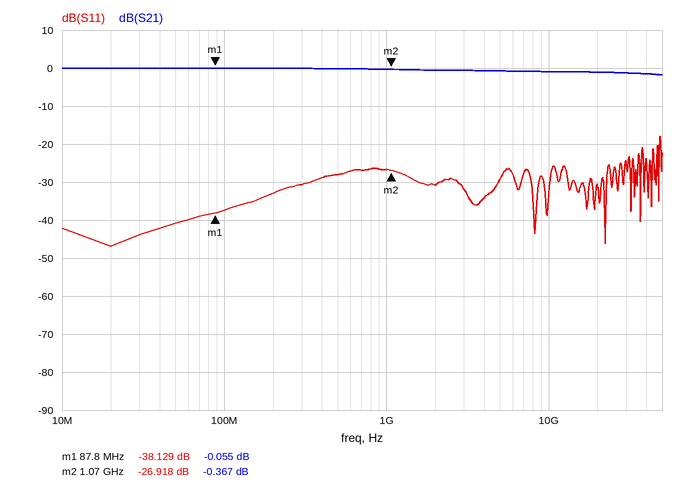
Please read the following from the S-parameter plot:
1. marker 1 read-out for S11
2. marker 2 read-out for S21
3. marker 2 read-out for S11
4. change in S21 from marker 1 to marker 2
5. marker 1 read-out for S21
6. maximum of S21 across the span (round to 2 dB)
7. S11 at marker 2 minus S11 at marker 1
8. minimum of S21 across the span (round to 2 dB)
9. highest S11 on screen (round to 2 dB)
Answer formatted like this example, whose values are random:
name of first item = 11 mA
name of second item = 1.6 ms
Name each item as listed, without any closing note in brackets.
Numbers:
marker 1 read-out for S11 = -38.129 dB
marker 2 read-out for S21 = -0.367 dB
marker 2 read-out for S11 = -26.918 dB
change in S21 from marker 1 to marker 2 = -0.312 dB
marker 1 read-out for S21 = -0.055 dB
maximum of S21 across the span = 0 dB
S11 at marker 2 minus S11 at marker 1 = 11.211 dB
minimum of S21 across the span = -2 dB
highest S11 on screen = -18 dB
